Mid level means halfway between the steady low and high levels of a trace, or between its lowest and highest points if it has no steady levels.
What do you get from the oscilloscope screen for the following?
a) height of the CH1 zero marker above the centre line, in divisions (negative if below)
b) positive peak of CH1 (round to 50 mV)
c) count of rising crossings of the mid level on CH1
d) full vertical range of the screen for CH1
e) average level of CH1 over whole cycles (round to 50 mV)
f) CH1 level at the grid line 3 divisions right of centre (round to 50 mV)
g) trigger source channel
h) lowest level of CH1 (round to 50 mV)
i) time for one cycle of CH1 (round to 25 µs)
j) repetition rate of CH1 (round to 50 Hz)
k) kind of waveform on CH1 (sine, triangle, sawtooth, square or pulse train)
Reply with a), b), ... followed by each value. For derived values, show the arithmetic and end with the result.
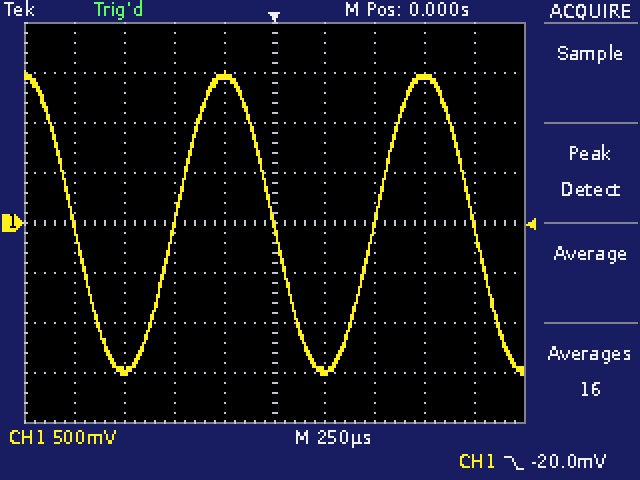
a) 0.0 div
b) 1.50 V
c) 2
d) 4 V
e) (1.50 V + (-1.50 V)) / 2 ≈ 0 mV
f) 1.45 V
g) CH1
h) -1.50 V
i) 1.000 ms
j) 1 / 1.000 ms ≈ 1.00 kHz
k) sine
